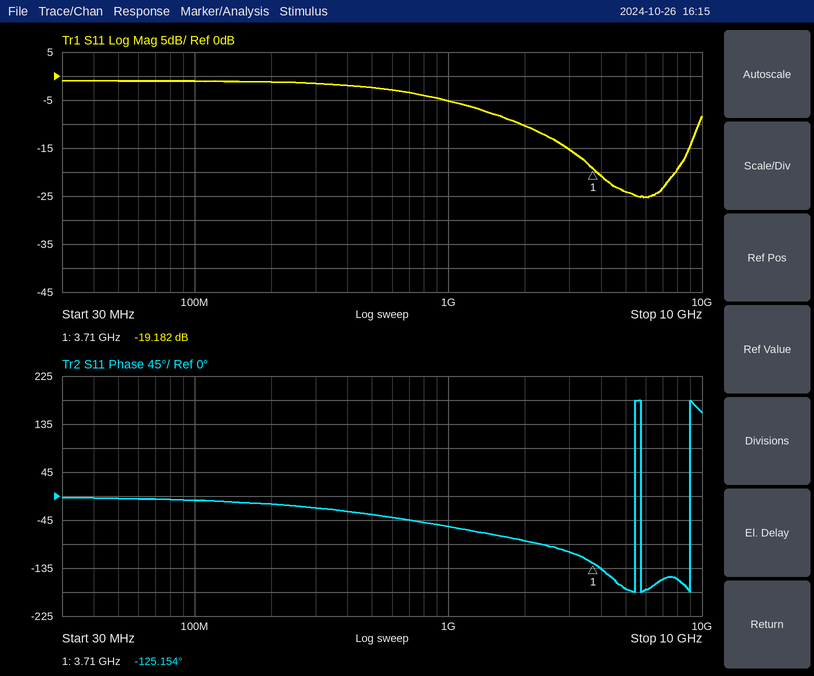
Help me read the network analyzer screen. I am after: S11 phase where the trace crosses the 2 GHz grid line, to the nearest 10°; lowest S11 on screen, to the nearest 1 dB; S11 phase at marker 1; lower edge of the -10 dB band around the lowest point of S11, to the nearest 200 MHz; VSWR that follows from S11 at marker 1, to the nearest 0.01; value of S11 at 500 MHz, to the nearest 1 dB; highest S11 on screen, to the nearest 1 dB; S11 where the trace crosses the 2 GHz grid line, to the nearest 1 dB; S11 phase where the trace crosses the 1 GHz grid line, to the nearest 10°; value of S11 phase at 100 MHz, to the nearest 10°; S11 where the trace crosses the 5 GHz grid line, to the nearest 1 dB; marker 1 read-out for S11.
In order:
-80°
-25 dB
-125.154°
2.0 GHz
1.25
-2 dB
-1 dB
-10 dB
-60°
-10°
-24 dB
-19.182 dB
